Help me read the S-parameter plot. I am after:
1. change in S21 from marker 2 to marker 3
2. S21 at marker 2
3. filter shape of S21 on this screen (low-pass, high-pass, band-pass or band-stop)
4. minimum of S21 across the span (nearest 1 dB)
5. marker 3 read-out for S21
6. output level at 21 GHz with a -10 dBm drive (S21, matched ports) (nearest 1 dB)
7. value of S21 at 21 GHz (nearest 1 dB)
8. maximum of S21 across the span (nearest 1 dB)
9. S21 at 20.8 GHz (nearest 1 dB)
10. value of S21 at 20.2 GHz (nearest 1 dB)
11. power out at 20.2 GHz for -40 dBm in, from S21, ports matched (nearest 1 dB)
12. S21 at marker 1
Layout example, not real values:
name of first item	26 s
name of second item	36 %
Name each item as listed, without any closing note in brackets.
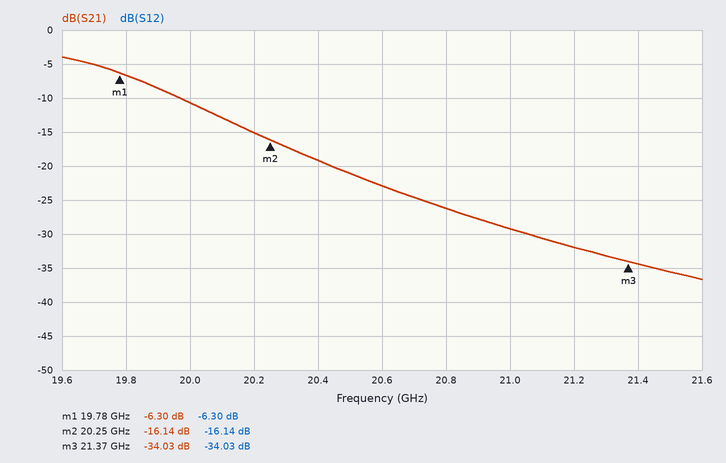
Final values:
change in S21 from marker 2 to marker 3	-17.89 dB
S21 at marker 2	-16.14 dB
filter shape of S21 on this screen	low-pass
minimum of S21 across the span	-37 dB
marker 3 read-out for S21	-34.03 dB
output level at 21 GHz with a -10 dBm drive (S21, matched ports)	-39 dBm
value of S21 at 21 GHz	-29 dB
maximum of S21 across the span	-4 dB
S21 at 20.8 GHz	-26 dB
value of S21 at 20.2 GHz	-15 dB
power out at 20.2 GHz for -40 dBm in, from S21, ports matched	-55 dBm
S21 at marker 1	-6.30 dB
